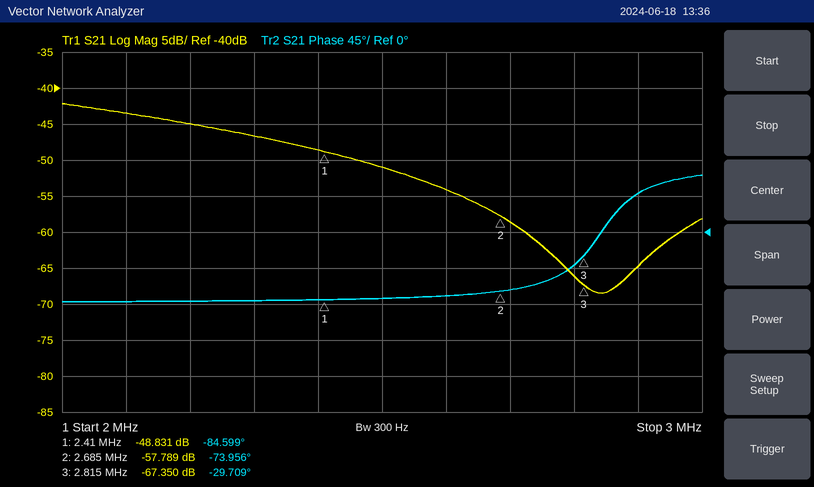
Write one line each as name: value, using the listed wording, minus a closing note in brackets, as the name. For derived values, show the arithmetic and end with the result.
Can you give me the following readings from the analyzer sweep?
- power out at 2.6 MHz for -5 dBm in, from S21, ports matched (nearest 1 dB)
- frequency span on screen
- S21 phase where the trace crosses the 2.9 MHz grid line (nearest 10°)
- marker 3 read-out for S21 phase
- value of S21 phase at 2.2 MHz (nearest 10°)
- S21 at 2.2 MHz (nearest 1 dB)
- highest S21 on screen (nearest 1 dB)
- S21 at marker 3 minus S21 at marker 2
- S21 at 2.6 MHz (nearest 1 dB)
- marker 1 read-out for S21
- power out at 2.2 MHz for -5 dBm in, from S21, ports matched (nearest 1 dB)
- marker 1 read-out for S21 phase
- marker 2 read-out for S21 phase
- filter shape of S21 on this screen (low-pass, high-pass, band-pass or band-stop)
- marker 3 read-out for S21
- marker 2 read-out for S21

power out at 2.6 MHz for -5 dBm in, from S21, ports matched: -5 dBm + (-54 dB) = -59 dBm
frequency span on screen: 1 MHz
S21 phase where the trace crosses the 2.9 MHz grid line: 50°
marker 3 read-out for S21 phase: -29.709°
value of S21 phase at 2.2 MHz: -90°
S21 at 2.2 MHz: -45 dB
highest S21 on screen: -42 dB
S21 at marker 3 minus S21 at marker 2: -67.35 − (-57.789) = -9.561 dB
S21 at 2.6 MHz: -54 dB
marker 1 read-out for S21: -48.831 dB
power out at 2.2 MHz for -5 dBm in, from S21, ports matched: -5 dBm + (-45 dB) = -50 dBm
marker 1 read-out for S21 phase: -84.599°
marker 2 read-out for S21 phase: -73.956°
filter shape of S21 on this screen: low-pass
marker 3 read-out for S21: -67.350 dB
marker 2 read-out for S21: -57.789 dB
